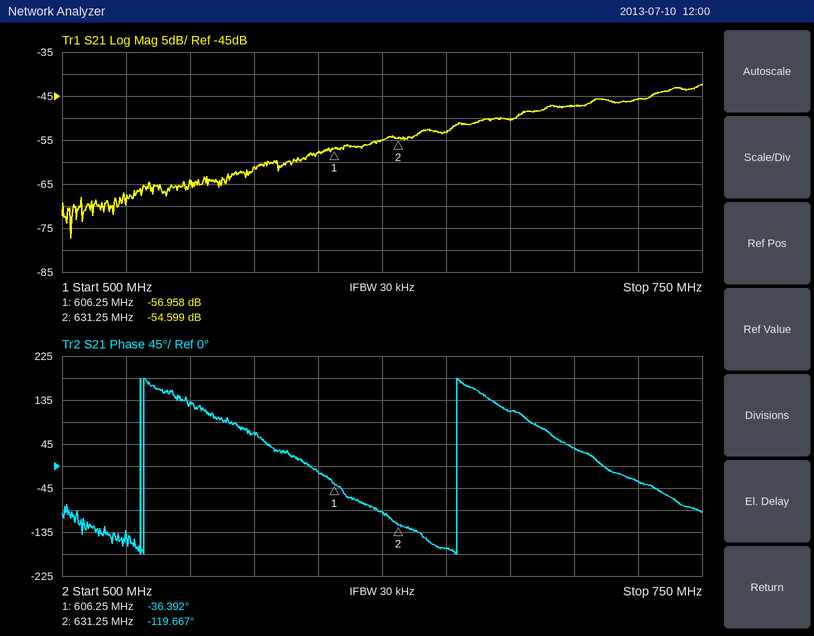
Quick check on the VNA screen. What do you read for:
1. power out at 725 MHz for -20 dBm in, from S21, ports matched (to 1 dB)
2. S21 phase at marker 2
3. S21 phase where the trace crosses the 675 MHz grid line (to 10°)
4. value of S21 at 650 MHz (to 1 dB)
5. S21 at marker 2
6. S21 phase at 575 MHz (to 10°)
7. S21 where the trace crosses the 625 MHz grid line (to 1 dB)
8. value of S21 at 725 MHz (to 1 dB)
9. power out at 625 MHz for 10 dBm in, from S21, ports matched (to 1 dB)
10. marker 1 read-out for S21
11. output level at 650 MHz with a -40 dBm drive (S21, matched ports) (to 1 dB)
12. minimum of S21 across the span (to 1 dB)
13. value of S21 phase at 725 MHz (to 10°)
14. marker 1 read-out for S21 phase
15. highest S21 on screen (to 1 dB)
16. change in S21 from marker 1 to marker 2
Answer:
-66 dBm
-119.667°
110°
-53 dB
-54.599 dB
70°
-55 dB
-46 dB
-45 dBm
-56.958 dB
-93 dBm
-77 dB
-30°
-36.392°
-42 dB
2.359 dB
